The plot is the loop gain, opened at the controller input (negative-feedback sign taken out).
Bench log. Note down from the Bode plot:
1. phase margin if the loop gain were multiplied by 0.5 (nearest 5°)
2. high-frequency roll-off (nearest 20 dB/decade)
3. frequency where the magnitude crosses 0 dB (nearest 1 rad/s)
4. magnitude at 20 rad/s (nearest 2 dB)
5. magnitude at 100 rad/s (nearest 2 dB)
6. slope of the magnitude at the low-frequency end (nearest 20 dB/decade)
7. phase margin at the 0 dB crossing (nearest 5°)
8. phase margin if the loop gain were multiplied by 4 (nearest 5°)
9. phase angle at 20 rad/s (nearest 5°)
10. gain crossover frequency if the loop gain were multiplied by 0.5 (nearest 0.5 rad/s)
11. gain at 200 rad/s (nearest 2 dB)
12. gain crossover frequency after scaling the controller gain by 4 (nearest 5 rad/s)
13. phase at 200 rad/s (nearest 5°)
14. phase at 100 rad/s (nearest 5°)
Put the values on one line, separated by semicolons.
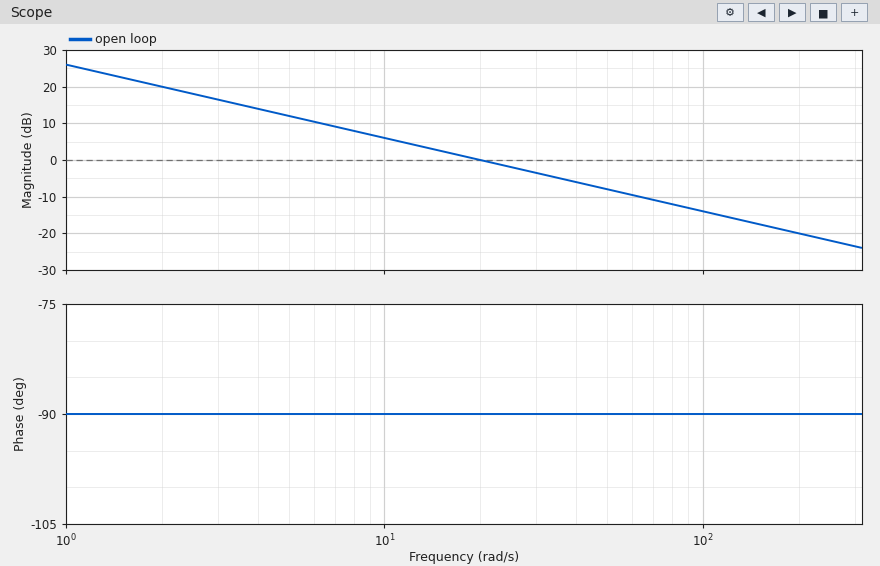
90°; -20 dB/decade; 20 rad/s; 0 dB; -14 dB; -20 dB/decade; 90°; 90°; -90°; 10.0 rad/s; -20 dB; 80 rad/s; -90°; -90°
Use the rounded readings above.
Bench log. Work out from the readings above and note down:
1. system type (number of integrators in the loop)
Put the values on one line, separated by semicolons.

1
